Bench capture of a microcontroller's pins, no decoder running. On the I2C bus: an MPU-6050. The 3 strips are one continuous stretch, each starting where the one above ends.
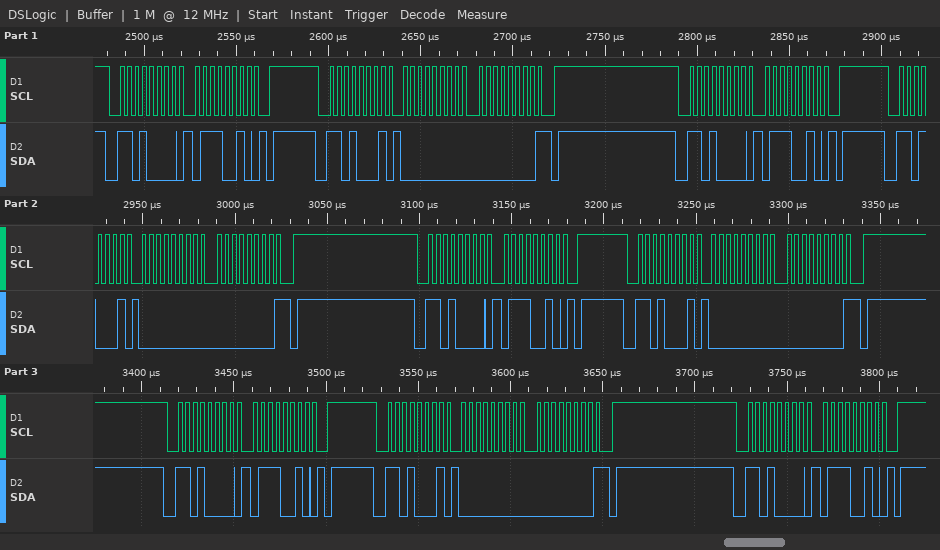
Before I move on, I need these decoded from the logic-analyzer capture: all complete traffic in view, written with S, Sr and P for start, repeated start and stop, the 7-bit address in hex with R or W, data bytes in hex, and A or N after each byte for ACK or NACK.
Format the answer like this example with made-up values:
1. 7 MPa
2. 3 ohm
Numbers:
1. S 68W A 72 A P S 68R A 00 A 00 N P S 68W A 72 A P S 68R A 00 A 00 N P S 68W A 72 A P S 68R A 00 A 00 N P S 68W A 72 A P S 68R A 00 A 00 N P S 68W A 72 A P
